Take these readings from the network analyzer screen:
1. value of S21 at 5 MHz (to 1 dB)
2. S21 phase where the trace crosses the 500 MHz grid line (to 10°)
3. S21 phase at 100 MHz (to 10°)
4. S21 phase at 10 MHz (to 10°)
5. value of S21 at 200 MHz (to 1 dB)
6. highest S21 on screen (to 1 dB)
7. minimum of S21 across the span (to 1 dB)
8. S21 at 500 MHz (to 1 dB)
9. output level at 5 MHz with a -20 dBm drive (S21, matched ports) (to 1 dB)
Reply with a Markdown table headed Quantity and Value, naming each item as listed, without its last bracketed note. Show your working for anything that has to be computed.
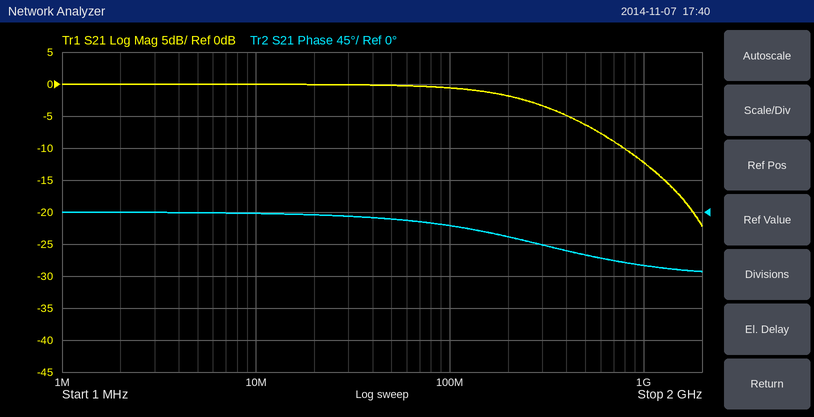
| Quantity | Value |
|---|---|
| value of S21 at 5 MHz | 0 dB |
| S21 phase where the trace crosses the 500 MHz grid line | -60° |
| S21 phase at 100 MHz | -20° |
| S21 phase at 10 MHz | 0° |
| value of S21 at 200 MHz | -2 dB |
| highest S21 on screen | 0 dB |
| minimum of S21 across the span | -22 dB |
| S21 at 500 MHz | -6 dB |
| output level at 5 MHz with a -20 dBm drive (S21, matched ports) | -20 dBm + (0 dB) = -20 dBm |
